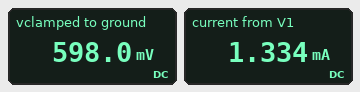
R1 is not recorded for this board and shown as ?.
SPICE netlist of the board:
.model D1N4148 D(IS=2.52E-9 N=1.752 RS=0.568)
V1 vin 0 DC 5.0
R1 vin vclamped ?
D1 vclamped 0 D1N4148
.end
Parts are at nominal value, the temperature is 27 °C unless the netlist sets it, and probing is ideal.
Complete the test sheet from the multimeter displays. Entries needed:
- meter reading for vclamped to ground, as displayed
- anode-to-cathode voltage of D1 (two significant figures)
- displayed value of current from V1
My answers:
598.0 mV
600 mV
1.334 mA
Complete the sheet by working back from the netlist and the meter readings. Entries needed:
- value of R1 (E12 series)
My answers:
3.3 kΩ
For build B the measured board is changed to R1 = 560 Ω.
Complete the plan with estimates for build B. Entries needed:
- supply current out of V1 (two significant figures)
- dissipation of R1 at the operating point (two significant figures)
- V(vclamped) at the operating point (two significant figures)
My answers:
7.7 mA
33 mW
680 mV
